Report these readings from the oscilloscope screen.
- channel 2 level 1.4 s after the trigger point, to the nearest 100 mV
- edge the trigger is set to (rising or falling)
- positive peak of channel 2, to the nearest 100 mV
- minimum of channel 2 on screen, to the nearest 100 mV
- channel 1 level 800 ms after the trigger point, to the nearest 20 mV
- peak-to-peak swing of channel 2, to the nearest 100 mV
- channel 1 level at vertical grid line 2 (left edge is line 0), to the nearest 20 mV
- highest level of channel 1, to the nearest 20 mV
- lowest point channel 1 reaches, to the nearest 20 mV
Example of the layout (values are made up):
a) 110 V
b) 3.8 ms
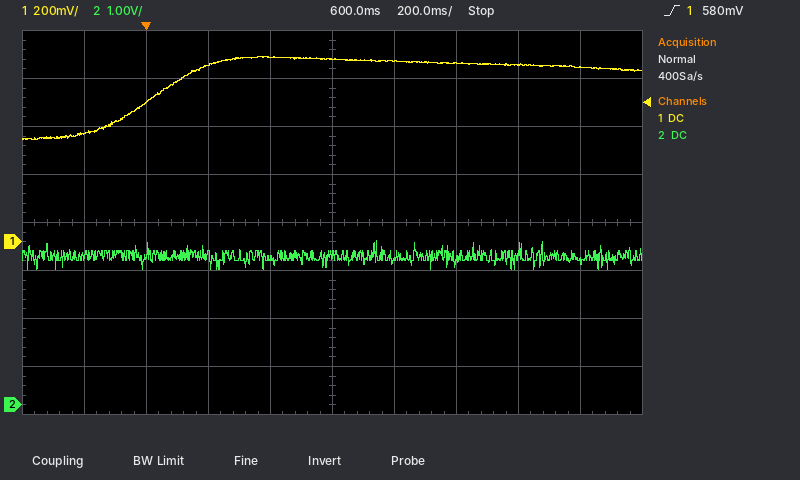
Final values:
a) 3.0 V
b) rising
c) 3.4 V
d) 2.8 V
e) 760 mV
f) 600 mV
g) 580 mV
h) 780 mV
i) 420 mV
